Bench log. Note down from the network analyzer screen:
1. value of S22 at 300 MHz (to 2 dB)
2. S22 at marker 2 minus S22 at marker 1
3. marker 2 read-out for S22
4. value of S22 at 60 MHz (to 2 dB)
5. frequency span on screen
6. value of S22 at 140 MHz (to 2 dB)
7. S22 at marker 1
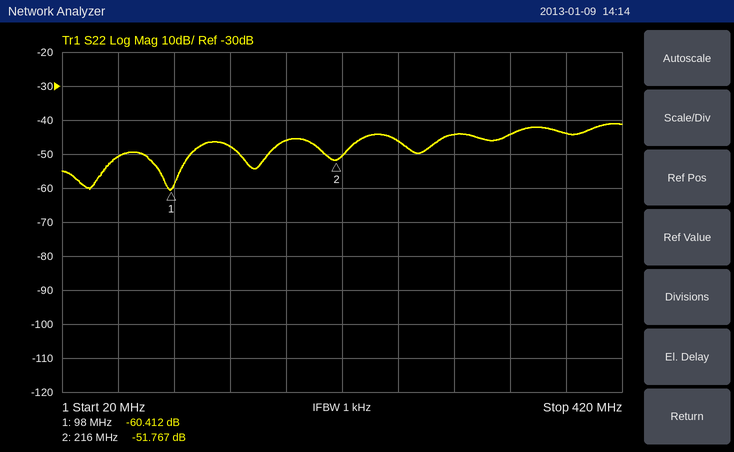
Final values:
-44 dB
8.645 dB
-51.767 dB
-50 dB
400 MHz
-48 dB
-60.412 dB
